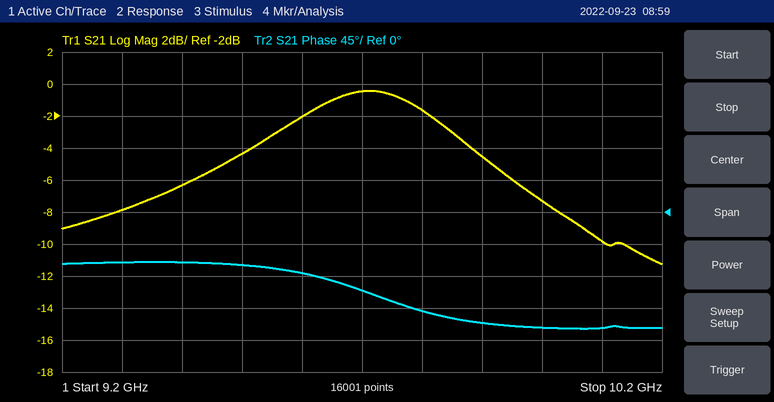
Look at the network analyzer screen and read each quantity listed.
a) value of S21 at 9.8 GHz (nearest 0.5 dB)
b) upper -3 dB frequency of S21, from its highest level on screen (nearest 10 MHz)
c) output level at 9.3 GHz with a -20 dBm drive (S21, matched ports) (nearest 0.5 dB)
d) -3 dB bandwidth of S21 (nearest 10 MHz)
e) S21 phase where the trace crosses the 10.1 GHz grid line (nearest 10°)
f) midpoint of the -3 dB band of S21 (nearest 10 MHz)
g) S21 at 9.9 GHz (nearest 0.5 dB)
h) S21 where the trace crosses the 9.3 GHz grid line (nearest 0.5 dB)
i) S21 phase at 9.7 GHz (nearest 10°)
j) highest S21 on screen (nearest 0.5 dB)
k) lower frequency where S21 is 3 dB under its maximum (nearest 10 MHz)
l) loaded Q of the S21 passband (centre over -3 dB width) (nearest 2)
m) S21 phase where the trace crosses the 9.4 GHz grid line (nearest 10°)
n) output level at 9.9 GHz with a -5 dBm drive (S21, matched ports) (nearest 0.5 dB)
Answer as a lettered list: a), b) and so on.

a) -1.5 dB
b) 9.86 GHz
c) -28.0 dBm
d) 320 MHz
e) -160°
f) 9.70 GHz
g) -4.5 dB
h) -8.0 dB
i) -110°
j) -0.5 dB
k) 9.54 GHz
l) 30
m) -70°
n) -9.5 dBm
